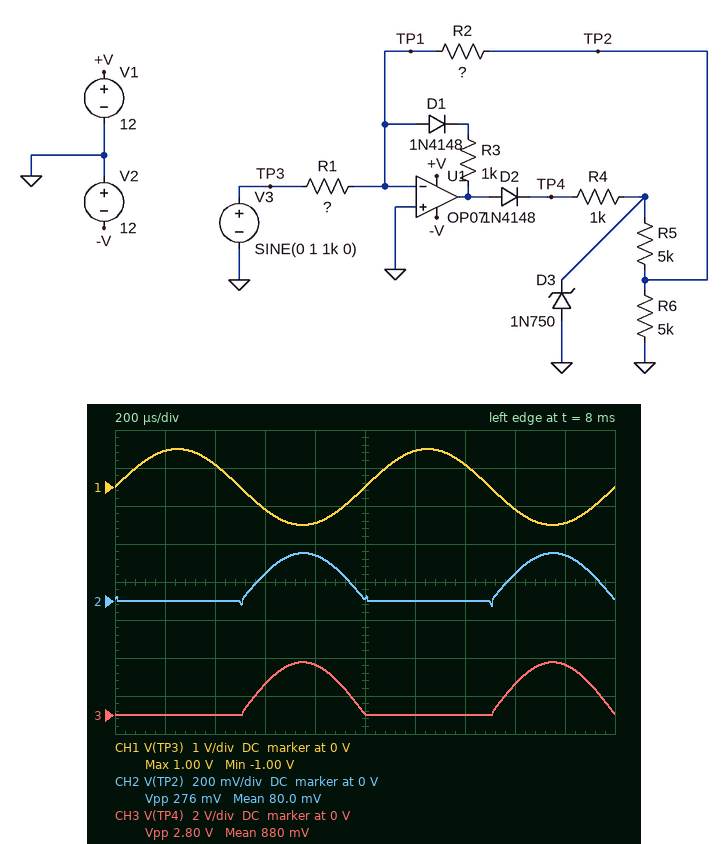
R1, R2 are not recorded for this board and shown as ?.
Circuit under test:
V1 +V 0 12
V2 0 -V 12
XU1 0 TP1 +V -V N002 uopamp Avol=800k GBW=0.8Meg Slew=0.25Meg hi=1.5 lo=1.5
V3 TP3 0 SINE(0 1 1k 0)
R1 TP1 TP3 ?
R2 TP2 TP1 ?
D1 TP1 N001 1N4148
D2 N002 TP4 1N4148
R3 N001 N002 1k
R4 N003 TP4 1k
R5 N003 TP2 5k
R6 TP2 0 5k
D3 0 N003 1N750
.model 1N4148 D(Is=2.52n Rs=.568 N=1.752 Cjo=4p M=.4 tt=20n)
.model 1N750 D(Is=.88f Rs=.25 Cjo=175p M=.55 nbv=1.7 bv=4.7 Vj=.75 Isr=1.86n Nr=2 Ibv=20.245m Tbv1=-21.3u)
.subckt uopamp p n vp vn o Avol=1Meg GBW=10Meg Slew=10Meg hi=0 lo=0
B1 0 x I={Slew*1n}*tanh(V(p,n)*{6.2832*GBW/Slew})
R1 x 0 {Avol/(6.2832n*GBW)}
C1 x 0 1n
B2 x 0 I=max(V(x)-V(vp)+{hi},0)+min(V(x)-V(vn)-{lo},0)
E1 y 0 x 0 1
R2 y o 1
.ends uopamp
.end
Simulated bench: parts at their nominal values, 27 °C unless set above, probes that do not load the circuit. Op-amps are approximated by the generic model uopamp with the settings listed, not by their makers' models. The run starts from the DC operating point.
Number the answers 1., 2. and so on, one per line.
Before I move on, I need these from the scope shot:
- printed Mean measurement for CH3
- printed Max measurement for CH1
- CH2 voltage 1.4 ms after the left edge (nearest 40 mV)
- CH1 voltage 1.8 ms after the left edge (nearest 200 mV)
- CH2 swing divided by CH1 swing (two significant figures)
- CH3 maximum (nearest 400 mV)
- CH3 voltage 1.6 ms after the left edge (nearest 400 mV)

1. 880 mV
2. 1.00 V
3. 0 V
4. -1.0 V
5. 0.14
6. 2.8 V
7. 1.6 V
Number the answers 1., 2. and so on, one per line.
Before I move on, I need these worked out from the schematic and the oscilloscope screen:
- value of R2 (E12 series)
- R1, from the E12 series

1. 680 Ω
2. 2.7 kΩ
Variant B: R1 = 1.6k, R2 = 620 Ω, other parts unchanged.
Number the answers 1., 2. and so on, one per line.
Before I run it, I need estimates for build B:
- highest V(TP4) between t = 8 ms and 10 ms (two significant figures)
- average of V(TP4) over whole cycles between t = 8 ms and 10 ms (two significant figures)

1. 4.6 V
2. 1.5 V
